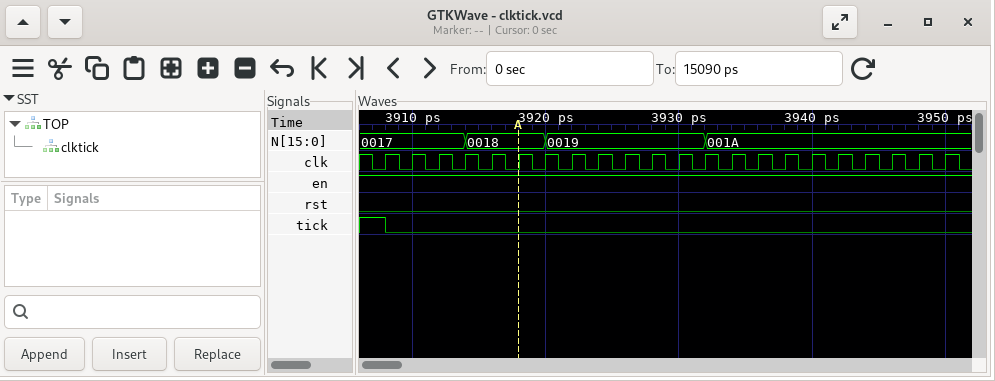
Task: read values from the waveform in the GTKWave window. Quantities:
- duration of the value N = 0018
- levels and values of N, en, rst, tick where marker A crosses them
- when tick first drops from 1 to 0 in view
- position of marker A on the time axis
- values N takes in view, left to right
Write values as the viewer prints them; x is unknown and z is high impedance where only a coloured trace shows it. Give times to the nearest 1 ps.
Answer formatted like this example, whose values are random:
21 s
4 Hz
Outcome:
6 ps
N=0018, en=1, rst=0, tick=0
3908 ps
3918 ps
0017, 0018, 0019, 001A
